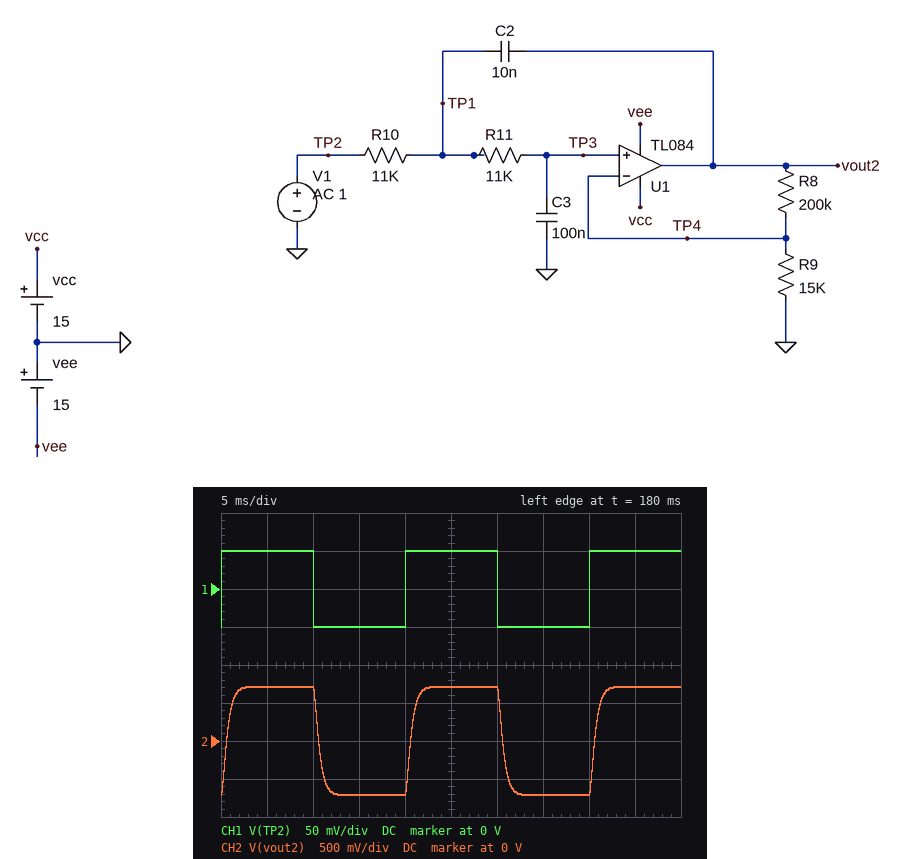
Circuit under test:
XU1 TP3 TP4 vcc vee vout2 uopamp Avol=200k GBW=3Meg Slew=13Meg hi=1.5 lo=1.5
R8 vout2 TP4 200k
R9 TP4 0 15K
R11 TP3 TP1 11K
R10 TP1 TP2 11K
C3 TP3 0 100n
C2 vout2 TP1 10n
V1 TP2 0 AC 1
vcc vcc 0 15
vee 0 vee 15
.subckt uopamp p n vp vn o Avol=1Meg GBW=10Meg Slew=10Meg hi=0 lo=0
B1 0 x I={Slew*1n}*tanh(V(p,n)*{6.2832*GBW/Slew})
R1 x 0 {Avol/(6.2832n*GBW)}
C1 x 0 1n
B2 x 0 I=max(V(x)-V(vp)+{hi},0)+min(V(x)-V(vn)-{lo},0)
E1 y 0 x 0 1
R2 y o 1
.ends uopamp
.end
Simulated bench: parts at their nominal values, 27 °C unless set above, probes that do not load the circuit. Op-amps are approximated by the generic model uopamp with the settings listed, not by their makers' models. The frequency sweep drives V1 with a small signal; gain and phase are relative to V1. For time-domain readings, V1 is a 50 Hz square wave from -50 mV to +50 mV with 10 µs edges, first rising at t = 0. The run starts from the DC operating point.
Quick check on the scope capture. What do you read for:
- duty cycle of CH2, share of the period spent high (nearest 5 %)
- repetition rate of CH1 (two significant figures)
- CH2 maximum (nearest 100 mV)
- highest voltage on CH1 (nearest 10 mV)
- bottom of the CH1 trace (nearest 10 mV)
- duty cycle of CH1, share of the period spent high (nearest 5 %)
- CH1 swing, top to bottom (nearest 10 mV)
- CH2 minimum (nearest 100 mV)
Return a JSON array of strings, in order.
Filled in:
["50 %", "50 Hz", "700 mV", "50 mV", "-50 mV", "50 %", "100 mV", "-700 mV"]
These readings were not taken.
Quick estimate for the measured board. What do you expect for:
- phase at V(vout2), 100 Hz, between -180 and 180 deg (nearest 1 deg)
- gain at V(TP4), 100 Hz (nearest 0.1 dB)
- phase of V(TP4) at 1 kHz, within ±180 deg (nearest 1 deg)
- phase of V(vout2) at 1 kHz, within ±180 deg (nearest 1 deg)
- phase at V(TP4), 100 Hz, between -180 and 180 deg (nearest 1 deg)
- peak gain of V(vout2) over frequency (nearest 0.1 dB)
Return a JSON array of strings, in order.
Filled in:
["-26 deg", "-0.5 dB", "-130 deg", "-130 deg", "-26 deg", "23.1 dB"]
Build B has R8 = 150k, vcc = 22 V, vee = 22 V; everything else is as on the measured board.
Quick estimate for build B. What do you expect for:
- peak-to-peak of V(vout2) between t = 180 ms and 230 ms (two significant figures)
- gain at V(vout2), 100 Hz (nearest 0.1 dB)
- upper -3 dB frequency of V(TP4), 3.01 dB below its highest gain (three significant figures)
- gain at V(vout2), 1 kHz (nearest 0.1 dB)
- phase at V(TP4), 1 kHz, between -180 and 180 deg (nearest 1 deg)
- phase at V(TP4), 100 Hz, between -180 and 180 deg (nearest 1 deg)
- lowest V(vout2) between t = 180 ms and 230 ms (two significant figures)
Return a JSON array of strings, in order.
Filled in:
["1.1 V", "19.4 dB", "161 Hz", "2.9 dB", "-119 deg", "-36 deg", "-550 mV"]
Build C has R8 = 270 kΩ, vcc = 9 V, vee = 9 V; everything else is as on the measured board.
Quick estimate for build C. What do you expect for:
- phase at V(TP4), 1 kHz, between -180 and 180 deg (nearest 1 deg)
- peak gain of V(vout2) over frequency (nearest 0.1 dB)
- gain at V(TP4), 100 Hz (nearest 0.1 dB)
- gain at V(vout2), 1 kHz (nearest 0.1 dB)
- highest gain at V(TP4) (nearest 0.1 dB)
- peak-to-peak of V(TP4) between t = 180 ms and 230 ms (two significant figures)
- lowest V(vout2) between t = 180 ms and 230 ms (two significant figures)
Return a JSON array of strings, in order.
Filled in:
["-161 deg", "30.1 dB", "0.3 dB", "13.3 dB", "4.5 dB", "170 mV", "-1.6 V"]
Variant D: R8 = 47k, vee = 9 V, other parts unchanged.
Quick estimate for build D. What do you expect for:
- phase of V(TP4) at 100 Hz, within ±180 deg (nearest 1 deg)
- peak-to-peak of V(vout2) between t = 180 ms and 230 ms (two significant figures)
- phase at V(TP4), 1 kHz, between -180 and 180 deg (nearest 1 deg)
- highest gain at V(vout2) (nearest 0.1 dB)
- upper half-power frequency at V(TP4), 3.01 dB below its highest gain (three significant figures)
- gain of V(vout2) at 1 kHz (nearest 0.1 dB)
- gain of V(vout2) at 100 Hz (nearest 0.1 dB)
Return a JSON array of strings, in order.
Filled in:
["-51 deg", "410 mV", "-108 deg", "12.3 dB", "88.9 Hz", "-9.4 dB", "8.8 dB"]
